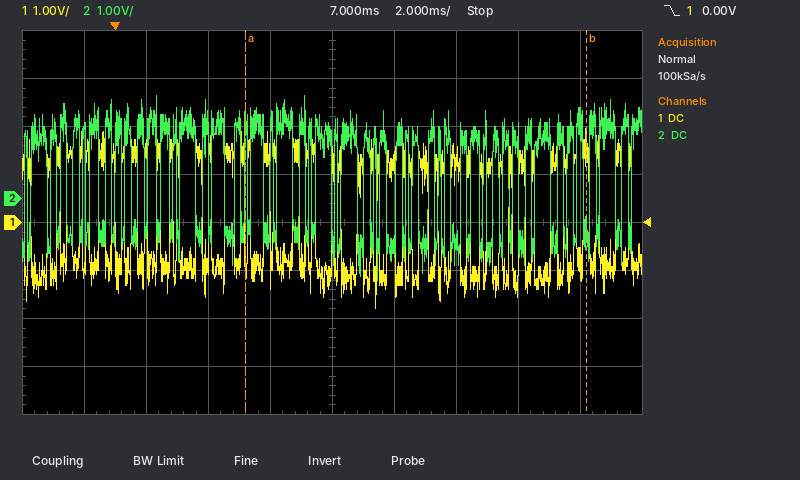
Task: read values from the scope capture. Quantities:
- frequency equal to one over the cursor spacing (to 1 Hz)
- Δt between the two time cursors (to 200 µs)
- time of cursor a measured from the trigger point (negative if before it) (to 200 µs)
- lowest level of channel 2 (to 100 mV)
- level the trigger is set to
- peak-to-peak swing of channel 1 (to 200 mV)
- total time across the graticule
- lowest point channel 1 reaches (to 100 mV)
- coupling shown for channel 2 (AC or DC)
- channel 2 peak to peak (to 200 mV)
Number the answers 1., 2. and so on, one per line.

1. 91 Hz
2. 11.0 ms
3. +4.2 ms
4. -1.7 V
5. 0.00 V
6. 3.8 V
7. 20 ms
8. -1.8 V
9. DC
10. 3.8 V
